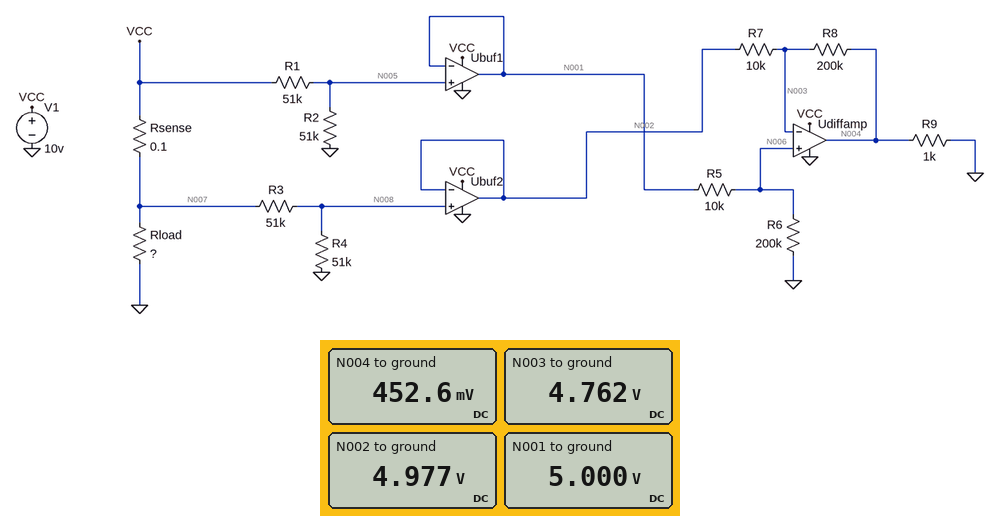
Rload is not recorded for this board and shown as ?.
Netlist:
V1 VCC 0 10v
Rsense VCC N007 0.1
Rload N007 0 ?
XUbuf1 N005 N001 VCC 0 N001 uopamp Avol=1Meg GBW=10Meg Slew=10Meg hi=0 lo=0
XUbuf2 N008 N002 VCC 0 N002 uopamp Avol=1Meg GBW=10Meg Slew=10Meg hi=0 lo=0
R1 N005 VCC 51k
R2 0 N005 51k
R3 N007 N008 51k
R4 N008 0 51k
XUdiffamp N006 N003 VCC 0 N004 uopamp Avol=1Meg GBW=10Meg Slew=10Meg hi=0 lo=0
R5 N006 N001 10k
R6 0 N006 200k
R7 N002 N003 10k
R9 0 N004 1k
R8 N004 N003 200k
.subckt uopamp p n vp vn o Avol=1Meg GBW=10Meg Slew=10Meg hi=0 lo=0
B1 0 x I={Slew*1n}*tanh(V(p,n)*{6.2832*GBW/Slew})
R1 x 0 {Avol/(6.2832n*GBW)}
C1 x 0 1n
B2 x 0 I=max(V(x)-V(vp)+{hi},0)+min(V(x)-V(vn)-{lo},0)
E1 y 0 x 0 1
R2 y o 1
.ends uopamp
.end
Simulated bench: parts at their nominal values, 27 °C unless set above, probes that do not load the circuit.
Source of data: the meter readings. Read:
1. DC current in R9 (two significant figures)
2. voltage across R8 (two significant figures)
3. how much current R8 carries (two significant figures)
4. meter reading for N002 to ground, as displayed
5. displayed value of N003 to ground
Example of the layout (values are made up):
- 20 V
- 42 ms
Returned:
- 450 µA
- 4.3 V
- 22 µA
- 4.977 V
- 4.762 V
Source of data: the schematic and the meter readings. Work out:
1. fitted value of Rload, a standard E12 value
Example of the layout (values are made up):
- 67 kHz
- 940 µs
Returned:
- 22 Ω
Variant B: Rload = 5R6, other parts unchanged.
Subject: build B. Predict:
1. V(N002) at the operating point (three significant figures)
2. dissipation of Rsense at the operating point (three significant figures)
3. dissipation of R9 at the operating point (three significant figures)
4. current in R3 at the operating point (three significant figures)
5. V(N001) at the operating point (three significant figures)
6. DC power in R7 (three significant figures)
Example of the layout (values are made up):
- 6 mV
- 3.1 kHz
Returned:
- 4.91 V
- 308 mW
- 3.08 mW
- 96.3 µA
- 5.00 V
- 2.26 µW
